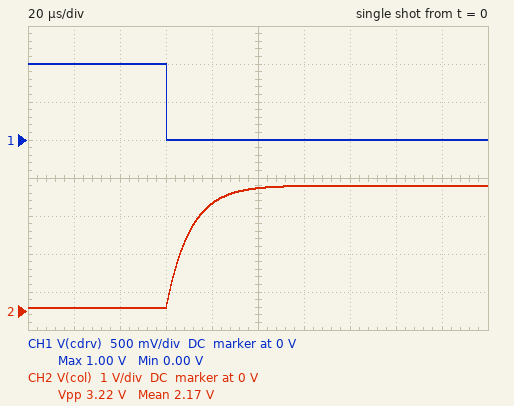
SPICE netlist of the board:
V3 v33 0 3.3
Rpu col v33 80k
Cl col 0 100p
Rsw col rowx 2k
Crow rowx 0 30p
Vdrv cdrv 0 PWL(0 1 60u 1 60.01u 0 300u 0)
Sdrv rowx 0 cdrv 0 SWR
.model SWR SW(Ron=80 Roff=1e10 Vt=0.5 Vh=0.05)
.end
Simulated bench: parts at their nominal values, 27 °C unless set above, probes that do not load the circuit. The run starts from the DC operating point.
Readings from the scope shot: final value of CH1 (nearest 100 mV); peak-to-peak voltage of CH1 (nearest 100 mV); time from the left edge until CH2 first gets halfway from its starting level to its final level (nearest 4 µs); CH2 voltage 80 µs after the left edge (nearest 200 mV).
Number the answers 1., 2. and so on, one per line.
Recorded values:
1. 0 V
2. 1.0 V
3. 68 µs
4. 2.8 V
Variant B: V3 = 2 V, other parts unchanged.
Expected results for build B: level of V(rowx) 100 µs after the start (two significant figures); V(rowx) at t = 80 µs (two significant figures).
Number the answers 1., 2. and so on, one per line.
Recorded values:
1. 2.0 V
2. 1.7 V
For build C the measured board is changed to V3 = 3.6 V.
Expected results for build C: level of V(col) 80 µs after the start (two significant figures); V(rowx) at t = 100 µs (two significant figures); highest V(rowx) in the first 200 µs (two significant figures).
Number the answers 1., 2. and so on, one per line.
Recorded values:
1. 3.1 V
2. 3.5 V
3. 3.6 V
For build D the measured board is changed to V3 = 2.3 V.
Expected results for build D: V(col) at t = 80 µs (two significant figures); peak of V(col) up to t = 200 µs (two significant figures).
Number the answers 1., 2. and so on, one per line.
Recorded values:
1. 2.0 V
2. 2.3 V
